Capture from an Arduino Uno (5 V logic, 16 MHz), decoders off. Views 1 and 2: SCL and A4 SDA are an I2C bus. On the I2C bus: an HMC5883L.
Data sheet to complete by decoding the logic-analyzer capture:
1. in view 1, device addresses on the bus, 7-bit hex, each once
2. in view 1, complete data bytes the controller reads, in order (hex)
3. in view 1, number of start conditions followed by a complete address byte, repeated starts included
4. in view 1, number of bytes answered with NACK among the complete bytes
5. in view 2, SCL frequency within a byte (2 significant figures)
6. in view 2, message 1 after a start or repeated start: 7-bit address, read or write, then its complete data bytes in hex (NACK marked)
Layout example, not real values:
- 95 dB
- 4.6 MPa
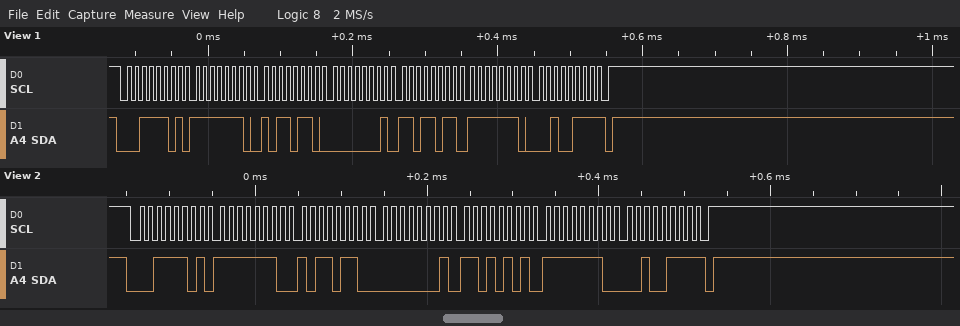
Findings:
- 0x1E
- FE B6 01 DB FE 27
- 1
- 1
- 100 kHz
- 0x1E read: FE B6 01 D5 FE 27 NACK
